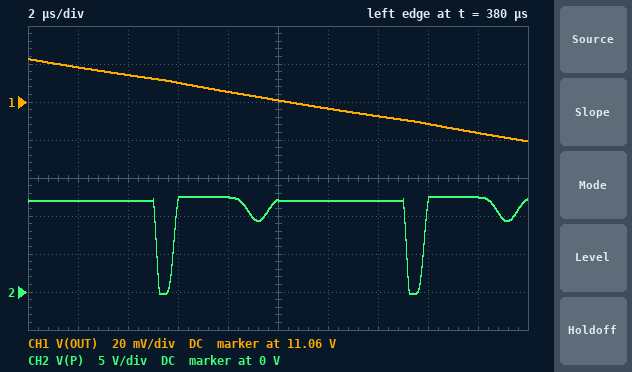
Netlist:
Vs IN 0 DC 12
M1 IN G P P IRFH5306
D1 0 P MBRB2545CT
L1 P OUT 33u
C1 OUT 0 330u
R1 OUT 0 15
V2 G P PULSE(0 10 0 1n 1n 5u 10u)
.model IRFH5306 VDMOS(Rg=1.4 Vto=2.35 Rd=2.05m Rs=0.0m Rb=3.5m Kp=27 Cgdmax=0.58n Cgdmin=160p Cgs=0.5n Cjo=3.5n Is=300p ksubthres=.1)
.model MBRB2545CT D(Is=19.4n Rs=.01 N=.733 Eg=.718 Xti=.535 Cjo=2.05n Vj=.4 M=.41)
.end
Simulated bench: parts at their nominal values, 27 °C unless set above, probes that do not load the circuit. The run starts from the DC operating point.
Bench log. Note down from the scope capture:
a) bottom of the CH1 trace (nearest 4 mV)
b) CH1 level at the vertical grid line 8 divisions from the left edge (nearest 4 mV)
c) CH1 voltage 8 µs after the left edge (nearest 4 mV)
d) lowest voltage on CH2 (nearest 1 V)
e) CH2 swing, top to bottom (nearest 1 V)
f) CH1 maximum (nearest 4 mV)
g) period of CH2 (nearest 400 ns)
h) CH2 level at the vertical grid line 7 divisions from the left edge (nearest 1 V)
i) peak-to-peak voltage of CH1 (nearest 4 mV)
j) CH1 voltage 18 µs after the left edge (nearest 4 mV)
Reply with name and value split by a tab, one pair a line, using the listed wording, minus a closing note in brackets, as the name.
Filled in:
bottom of the CH1 trace	11.040 V
CH1 level at the vertical grid line 8 divisions from the left edge	11.048 V
CH1 voltage 8 µs after the left edge	11.064 V
lowest voltage on CH2	0 V
CH2 swing, top to bottom	13 V
CH1 maximum	11.084 V
period of CH2	10.0 µs
CH2 level at the vertical grid line 7 divisions from the left edge	12 V
peak-to-peak voltage of CH1	44 mV
CH1 voltage 18 µs after the left edge	11.044 V
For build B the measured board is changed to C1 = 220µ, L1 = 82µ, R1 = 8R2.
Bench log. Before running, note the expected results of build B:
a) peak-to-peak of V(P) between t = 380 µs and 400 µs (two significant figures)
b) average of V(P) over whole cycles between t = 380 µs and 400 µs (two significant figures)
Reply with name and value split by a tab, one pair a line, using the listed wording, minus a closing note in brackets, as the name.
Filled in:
peak-to-peak of V(P) between t = 380 µs and 400 µs	12 V
average of V(P) over whole cycles between t = 380 µs and 400 µs	5.8 V
